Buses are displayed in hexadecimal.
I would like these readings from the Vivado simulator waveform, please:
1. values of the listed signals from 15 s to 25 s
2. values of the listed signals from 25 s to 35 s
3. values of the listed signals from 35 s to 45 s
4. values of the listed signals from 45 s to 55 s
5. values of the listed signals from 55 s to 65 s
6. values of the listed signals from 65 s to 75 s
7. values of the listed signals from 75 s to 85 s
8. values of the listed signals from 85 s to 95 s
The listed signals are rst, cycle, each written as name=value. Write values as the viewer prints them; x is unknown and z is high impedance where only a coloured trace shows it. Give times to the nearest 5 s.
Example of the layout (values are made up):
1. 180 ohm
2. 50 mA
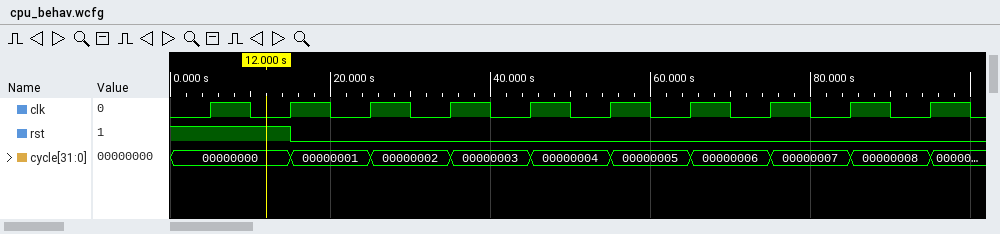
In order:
1. rst=0, cycle=00000001
2. rst=0, cycle=00000002
3. rst=0, cycle=00000003
4. rst=0, cycle=00000004
5. rst=0, cycle=00000005
6. rst=0, cycle=00000006
7. rst=0, cycle=00000007
8. rst=0, cycle=00000008
